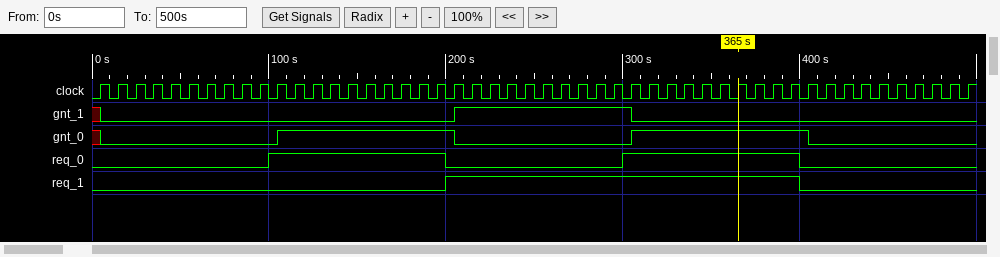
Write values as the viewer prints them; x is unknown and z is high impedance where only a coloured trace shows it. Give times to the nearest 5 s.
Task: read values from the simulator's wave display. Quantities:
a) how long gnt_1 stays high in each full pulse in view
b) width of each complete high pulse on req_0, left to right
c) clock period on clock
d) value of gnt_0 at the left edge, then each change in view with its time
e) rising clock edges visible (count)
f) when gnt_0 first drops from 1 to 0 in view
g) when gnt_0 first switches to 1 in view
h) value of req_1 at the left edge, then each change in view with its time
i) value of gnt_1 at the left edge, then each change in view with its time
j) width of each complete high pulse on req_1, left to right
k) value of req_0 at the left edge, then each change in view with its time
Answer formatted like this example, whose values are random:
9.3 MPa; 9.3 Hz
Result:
100 s; 100 s, 100 s; 10 s; x, 0 at 5 s, 1 at 105 s, 0 at 205 s, 1 at 305 s, 0 at 405 s; 50; 205 s; 105 s; 0, 1 at 200 s, 0 at 400 s; x, 0 at 5 s, 1 at 205 s, 0 at 305 s; 200 s; 0, 1 at 100 s, 0 at 200 s, 1 at 300 s, 0 at 400 s
